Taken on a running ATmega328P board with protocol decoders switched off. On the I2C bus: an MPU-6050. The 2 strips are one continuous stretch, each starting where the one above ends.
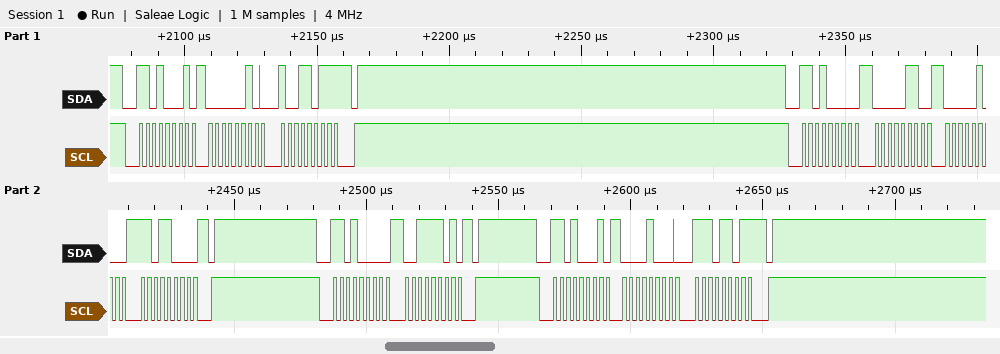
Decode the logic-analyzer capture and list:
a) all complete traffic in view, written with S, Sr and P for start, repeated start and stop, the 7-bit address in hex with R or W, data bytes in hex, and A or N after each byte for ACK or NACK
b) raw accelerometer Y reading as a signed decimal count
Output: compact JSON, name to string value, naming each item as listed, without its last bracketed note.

{"all complete traffic in view, written with S, Sr and P for start, repeated start and stop, the 7-bit address in hex with R or W, data bytes in hex, and A or N after each byte for ACK or NACK": "S 68R A 02 A 9B N P S 68W A 06 A 04 A D8 A P S 68W A 3D A P S 68R A 08 A ED N P", "raw accelerometer Y reading as a signed decimal count": "2285"}
